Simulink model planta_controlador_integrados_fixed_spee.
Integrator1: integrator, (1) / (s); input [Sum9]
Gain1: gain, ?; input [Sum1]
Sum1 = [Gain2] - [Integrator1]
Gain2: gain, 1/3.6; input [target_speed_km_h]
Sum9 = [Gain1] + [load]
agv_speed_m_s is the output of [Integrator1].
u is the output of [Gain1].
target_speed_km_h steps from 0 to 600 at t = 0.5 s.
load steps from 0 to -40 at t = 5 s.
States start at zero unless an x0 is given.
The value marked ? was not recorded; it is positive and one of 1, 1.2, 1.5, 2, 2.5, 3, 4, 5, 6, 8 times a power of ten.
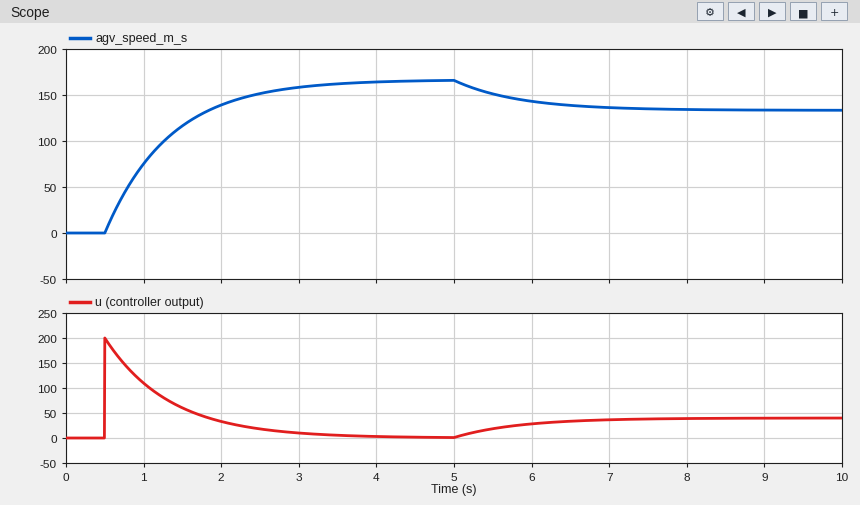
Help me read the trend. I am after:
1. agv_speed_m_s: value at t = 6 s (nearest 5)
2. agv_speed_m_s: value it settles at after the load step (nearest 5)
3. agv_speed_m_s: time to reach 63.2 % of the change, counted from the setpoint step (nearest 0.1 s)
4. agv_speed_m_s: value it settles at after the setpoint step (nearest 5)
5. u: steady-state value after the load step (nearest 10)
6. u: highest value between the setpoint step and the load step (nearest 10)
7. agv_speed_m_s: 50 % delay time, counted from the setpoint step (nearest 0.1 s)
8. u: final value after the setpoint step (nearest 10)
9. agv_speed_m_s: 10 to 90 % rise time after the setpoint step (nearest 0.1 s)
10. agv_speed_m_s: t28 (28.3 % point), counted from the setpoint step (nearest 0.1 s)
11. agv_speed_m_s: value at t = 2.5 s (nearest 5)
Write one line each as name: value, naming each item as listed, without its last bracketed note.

agv_speed_m_s: value at t = 6 s: 145
agv_speed_m_s: value it settles at after the load step: 135
agv_speed_m_s: time to reach 63.2 % of the change, counted from the setpoint step: 0.8 s
agv_speed_m_s: value it settles at after the setpoint step: 165
u: steady-state value after the load step: 40
u: highest value between the setpoint step and the load step: 200
agv_speed_m_s: 50 % delay time, counted from the setpoint step: 0.6 s
u: final value after the setpoint step: 0
agv_speed_m_s: 10 to 90 % rise time after the setpoint step: 1.8 s
agv_speed_m_s: t28 (28.3 % point), counted from the setpoint step: 0.3 s
agv_speed_m_s: value at t = 2.5 s: 150
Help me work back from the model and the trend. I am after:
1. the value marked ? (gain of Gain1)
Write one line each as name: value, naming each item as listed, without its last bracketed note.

the value marked ?: 1.2
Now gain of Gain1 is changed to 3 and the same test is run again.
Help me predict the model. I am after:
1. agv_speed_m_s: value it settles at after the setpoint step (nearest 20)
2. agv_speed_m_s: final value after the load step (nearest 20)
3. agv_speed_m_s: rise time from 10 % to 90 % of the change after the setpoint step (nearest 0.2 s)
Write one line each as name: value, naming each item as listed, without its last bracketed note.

agv_speed_m_s: value it settles at after the setpoint step: 160
agv_speed_m_s: final value after the load step: 160
agv_speed_m_s: rise time from 10 % to 90 % of the change after the setpoint step: 0.8 s
